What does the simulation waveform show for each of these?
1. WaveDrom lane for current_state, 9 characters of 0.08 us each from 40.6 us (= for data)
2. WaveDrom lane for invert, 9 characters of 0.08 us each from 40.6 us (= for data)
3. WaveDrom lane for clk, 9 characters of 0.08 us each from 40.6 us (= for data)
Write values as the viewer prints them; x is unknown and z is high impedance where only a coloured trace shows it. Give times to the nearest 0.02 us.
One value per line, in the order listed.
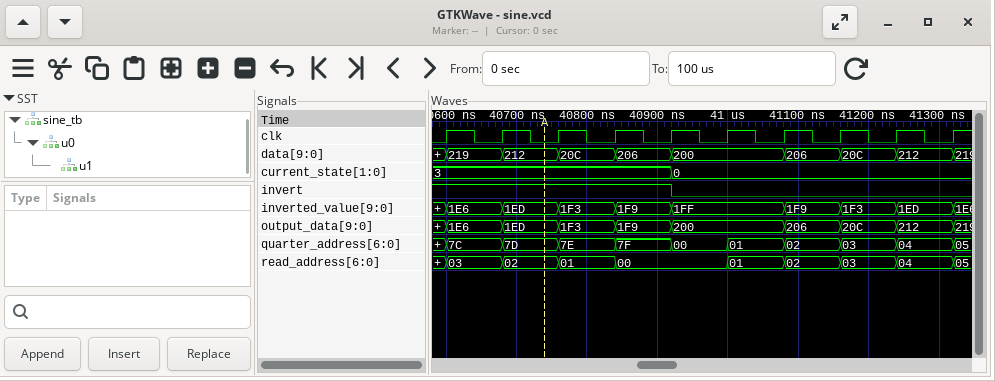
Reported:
{name: 'current_state', wave: '=...=....', data: '3 0'}
{name: 'invert', wave: '1...0....'}
{name: 'clk', wave: 'p........'}
